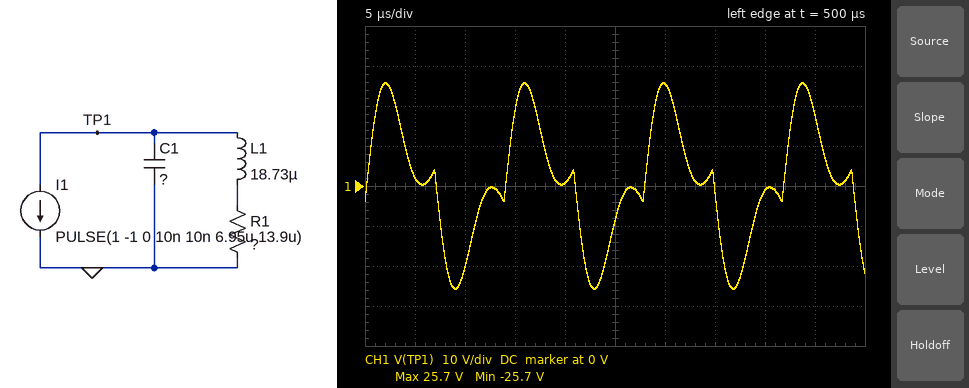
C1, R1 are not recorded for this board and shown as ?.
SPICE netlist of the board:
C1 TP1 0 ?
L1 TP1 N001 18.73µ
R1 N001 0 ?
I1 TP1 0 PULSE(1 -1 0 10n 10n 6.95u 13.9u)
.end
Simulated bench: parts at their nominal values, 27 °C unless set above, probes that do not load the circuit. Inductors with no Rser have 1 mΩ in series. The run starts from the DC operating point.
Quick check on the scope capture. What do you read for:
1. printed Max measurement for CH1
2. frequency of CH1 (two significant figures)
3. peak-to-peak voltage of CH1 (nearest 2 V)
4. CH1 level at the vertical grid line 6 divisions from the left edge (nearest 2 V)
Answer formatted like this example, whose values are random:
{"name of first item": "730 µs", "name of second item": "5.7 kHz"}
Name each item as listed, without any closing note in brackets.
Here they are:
{"printed Max measurement for CH1": "25.7 V", "frequency of CH1": "72 kHz", "peak-to-peak voltage of CH1": "52 V", "CH1 level at the vertical grid line 6 divisions from the left edge": "26 V"}
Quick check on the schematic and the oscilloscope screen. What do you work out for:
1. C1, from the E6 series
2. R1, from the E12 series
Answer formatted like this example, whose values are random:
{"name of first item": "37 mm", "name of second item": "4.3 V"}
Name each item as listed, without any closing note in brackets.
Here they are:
{"C1, from the E6 series": "68 nF", "R1, from the E12 series": "8.2 Ω"}
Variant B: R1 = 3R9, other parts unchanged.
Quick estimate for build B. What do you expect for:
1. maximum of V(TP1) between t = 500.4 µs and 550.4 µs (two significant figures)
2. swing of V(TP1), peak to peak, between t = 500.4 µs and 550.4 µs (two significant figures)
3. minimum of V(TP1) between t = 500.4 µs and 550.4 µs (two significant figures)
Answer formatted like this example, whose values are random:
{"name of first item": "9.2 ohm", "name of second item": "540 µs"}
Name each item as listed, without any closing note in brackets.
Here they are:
{"maximum of V(TP1) between t = 500.4 µs and 550.4 µs": "22 V", "swing of V(TP1), peak to peak, between t = 500.4 µs and 550.4 µs": "45 V", "minimum of V(TP1) between t = 500.4 µs and 550.4 µs": "-22 V"}
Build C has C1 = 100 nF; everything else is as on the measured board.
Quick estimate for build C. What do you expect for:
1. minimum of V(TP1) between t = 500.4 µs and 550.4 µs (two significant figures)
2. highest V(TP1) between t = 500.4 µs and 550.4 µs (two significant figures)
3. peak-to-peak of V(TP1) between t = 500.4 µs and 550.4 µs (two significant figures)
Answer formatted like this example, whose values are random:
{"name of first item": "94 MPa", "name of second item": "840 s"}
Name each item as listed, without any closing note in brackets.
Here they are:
{"minimum of V(TP1) between t = 500.4 µs and 550.4 µs": "-24 V", "highest V(TP1) between t = 500.4 µs and 550.4 µs": "24 V", "peak-to-peak of V(TP1) between t = 500.4 µs and 550.4 µs": "47 V"}
